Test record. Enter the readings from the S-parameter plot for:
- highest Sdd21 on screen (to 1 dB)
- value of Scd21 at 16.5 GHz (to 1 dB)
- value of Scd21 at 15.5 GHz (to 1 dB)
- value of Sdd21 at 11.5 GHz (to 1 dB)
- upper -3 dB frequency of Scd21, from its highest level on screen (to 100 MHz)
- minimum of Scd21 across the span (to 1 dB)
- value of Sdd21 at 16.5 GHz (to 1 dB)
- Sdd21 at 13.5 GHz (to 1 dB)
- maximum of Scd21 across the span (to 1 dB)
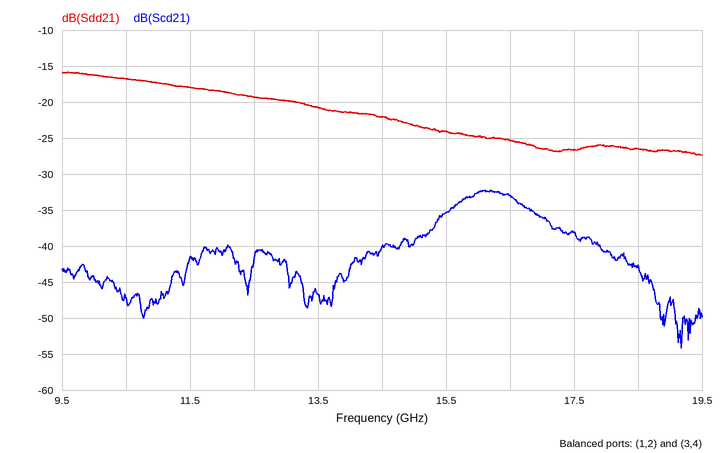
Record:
-16 dB
-33 dB
-35 dB
-18 dB
16.9 GHz
-54 dB
-25 dB
-21 dB
-32 dB
